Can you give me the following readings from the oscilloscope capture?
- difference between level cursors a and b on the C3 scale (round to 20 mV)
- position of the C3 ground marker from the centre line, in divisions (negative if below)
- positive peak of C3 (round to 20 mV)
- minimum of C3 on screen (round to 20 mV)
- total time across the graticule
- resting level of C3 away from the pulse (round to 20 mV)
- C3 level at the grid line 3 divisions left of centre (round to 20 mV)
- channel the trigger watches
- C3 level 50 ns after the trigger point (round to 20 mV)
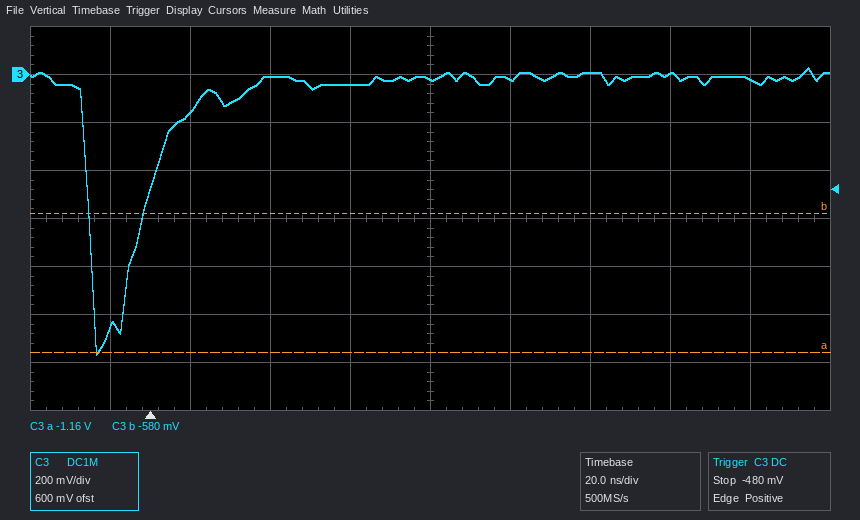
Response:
580 mV
+3.0 div
20 mV
-1.16 V
200 ns
-20 mV
-160 mV
C3
-40 mV
